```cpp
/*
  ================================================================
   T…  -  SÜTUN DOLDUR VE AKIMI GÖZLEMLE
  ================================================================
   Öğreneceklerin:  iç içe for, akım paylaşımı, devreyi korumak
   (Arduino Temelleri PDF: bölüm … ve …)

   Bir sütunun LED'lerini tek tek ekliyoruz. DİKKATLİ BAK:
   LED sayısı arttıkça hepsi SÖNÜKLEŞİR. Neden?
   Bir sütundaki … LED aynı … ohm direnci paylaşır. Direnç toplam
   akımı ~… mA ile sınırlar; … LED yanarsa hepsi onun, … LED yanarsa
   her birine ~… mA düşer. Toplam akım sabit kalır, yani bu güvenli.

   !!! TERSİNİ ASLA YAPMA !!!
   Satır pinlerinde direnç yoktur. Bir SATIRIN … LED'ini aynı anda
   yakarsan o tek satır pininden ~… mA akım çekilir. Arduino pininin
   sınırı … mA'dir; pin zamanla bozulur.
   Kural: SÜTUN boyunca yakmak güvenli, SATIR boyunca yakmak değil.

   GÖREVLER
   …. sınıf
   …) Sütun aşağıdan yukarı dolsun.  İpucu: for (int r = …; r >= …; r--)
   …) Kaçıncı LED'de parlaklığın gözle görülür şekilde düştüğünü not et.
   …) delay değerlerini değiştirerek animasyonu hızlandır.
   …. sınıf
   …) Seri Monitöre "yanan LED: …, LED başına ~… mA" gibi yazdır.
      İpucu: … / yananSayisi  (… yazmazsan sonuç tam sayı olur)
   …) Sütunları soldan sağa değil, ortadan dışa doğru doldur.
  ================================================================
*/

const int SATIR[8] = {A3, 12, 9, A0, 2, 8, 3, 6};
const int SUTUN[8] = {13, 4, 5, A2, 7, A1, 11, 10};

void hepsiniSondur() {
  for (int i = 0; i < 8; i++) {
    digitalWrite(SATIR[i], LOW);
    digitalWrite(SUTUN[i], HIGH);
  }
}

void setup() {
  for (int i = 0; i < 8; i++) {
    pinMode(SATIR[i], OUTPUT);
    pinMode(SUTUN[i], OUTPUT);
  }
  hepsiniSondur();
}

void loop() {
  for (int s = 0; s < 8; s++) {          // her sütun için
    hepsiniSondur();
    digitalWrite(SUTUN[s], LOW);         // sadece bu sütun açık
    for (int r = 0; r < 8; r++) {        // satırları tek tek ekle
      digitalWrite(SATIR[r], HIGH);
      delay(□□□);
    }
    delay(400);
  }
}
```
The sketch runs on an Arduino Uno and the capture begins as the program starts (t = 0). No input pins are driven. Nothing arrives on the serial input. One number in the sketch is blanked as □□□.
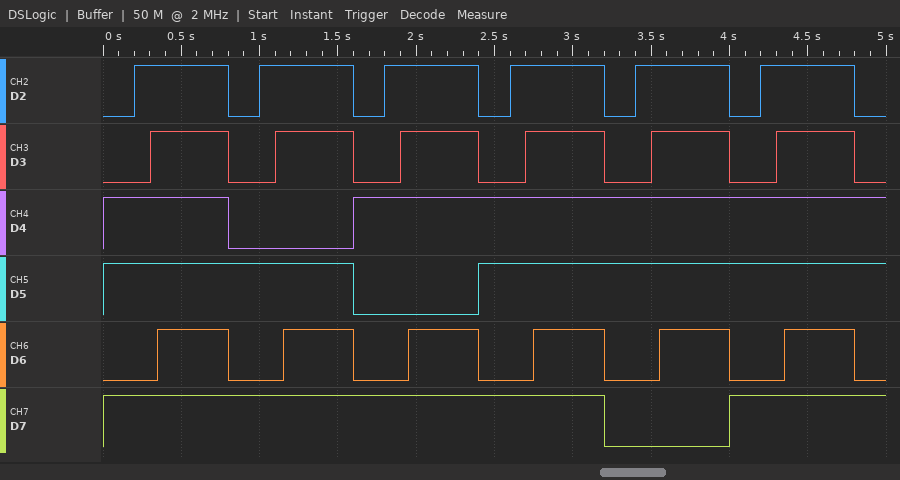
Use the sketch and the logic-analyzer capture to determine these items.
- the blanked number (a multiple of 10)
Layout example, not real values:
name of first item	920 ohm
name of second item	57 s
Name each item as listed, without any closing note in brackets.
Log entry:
the blanked number	50
